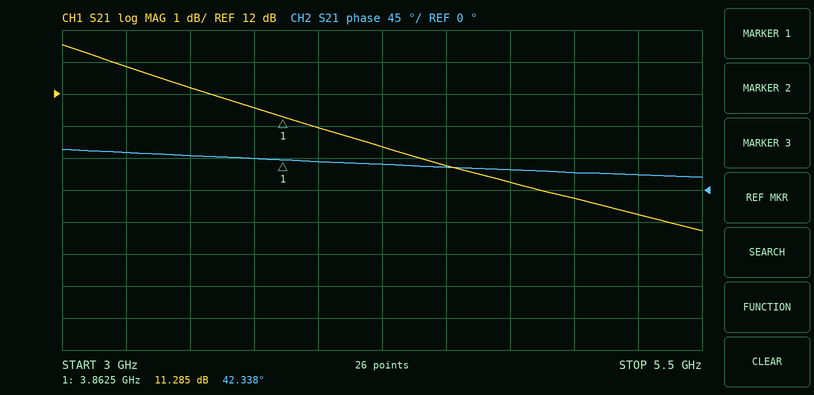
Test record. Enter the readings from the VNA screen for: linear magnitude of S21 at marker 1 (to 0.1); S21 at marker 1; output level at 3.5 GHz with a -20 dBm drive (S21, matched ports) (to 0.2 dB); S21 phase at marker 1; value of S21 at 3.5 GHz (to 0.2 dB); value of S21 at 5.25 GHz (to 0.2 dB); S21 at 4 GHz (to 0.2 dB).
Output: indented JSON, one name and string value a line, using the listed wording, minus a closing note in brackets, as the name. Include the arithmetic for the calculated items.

{
  "linear magnitude of S21 at marker 1": "10^(11.285/20) ≈ 3.7",
  "S21 at marker 1": "11.285 dB",
  "output level at 3.5 GHz with a -20 dBm drive (S21, matched ports)": "-20 dBm + (12.2 dB) = -7.8 dBm",
  "S21 phase at marker 1": "42.338°",
  "value of S21 at 3.5 GHz": "12.2 dB",
  "value of S21 at 5.25 GHz": "8.2 dB",
  "S21 at 4 GHz": "11.0 dB"
}
